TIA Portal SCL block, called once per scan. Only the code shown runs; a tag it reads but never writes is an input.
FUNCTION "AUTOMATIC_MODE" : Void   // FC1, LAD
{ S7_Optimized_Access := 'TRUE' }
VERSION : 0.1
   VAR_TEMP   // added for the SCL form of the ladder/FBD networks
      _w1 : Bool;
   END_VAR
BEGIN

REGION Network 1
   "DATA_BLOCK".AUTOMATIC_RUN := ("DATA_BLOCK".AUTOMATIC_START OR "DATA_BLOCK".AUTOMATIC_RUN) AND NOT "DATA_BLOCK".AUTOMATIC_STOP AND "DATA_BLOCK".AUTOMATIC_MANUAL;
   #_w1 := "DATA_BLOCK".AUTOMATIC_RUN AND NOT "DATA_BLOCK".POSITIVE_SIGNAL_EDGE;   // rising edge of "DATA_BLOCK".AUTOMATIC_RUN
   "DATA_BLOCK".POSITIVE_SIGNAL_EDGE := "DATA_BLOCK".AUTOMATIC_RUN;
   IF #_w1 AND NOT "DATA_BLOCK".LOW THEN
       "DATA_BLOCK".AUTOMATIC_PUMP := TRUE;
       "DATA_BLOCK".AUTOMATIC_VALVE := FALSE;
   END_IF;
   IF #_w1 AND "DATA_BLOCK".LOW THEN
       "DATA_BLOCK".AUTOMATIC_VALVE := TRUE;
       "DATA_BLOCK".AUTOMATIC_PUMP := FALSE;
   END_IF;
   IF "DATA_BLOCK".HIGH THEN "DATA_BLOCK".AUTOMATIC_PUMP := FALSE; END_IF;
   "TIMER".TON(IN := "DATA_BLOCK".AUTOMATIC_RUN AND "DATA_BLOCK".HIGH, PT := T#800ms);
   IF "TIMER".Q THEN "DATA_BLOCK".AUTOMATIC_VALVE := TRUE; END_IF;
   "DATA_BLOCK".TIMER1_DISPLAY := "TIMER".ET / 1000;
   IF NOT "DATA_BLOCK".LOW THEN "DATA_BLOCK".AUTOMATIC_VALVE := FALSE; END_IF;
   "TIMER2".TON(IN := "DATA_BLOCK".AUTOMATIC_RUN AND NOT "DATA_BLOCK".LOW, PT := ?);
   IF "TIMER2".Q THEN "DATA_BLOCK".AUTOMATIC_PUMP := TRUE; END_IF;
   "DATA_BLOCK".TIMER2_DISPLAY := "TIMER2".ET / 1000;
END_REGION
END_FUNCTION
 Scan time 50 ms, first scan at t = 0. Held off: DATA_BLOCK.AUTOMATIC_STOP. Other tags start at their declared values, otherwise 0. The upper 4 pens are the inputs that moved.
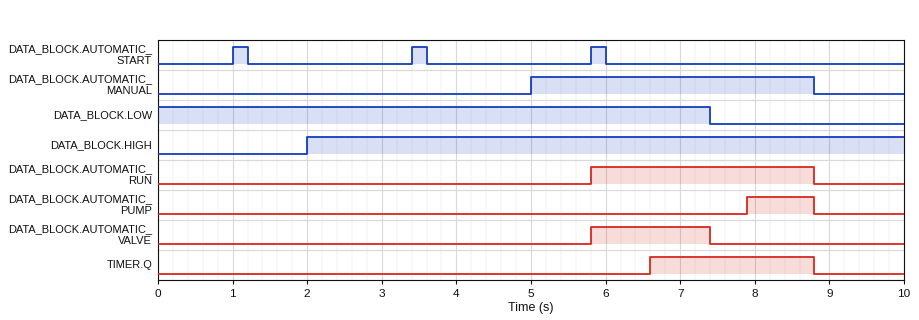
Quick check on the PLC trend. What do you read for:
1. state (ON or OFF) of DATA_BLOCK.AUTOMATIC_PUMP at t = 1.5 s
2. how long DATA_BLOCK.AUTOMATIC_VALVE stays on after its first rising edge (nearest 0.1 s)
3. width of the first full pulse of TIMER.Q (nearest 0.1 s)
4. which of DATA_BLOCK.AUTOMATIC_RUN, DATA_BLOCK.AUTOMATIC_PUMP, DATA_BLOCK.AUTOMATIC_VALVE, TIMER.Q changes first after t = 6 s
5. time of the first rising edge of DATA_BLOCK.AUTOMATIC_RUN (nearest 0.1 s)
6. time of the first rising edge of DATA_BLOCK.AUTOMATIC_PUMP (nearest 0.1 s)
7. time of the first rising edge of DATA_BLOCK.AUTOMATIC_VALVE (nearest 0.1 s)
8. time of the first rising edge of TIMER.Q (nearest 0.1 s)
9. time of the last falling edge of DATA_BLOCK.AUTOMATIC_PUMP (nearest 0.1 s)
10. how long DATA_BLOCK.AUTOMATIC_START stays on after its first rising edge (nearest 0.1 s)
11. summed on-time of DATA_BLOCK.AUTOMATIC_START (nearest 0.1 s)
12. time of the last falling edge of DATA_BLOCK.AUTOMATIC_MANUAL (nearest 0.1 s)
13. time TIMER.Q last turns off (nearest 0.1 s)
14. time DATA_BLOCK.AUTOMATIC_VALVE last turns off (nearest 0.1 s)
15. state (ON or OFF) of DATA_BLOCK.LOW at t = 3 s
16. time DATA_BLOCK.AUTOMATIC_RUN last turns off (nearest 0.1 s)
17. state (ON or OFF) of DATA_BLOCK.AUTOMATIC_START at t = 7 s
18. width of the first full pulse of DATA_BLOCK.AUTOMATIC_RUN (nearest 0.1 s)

OFF
1.6 s
2.2 s
TIMER.Q
5.8 s
7.9 s
5.8 s
6.6 s
8.8 s
0.2 s
0.6 s
8.8 s
8.8 s
7.4 s
ON
8.8 s
OFF
3.0 s
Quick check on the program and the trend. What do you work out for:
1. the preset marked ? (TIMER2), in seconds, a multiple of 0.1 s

0.5 s
